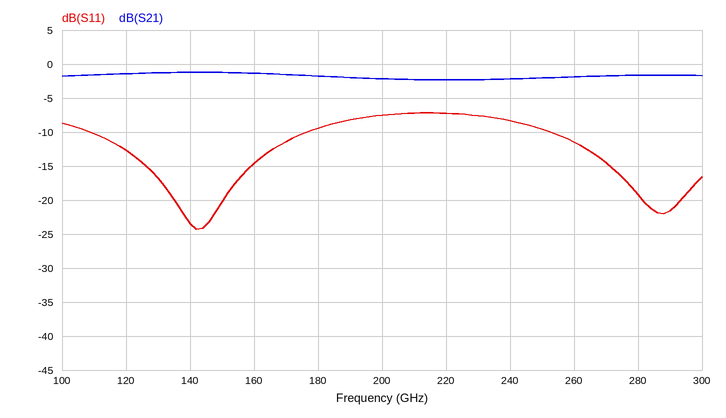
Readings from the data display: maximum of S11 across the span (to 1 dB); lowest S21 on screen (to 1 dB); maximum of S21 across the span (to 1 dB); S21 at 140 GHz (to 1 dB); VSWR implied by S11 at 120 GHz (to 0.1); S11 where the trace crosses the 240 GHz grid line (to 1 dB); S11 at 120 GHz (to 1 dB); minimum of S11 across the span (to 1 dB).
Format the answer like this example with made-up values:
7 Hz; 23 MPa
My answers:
-7 dB; -2 dB; -1 dB; -1 dB; 1.6; -8 dB; -13 dB; -24 dB
